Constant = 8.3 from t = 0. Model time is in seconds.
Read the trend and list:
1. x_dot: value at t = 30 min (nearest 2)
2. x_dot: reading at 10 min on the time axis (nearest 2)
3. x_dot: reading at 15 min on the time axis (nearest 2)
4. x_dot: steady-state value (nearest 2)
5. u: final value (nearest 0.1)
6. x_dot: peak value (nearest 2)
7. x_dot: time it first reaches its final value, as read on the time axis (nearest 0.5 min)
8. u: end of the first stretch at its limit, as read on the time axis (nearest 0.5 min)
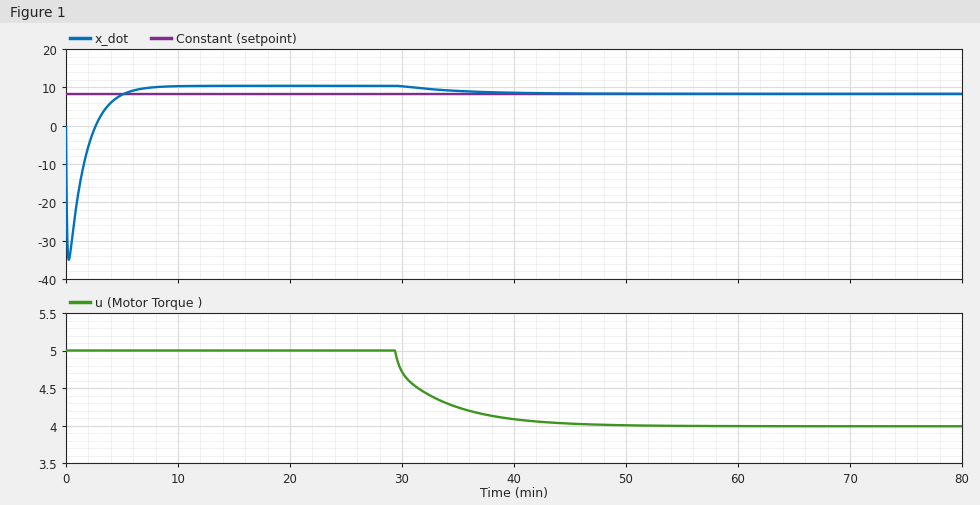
10
10
10
8
4.0
10
5.0 min
29.5 min
